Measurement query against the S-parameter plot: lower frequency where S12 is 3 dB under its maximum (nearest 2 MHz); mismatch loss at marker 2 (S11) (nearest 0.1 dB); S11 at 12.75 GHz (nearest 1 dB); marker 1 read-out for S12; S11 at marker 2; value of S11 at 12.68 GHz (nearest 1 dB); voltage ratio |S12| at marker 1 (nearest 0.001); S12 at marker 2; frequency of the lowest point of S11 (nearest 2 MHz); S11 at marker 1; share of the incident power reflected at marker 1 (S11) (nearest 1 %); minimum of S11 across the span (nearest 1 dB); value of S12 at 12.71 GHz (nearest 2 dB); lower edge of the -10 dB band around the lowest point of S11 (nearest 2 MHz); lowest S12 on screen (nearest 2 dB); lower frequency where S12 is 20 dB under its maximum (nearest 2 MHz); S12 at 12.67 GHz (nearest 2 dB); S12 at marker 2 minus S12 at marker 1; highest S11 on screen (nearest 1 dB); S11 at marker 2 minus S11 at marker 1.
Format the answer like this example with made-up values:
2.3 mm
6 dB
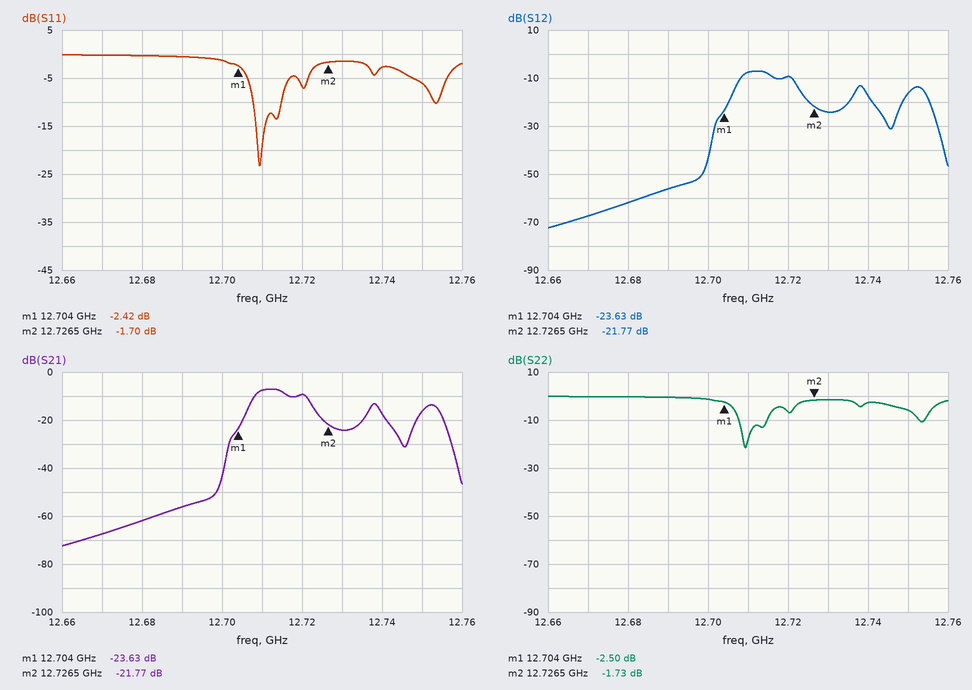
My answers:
12.708 GHz
4.9 dB
-6 dB
-23.63 dB
-1.70 dB
0 dB
0.066
-21.77 dB
12.710 GHz
-2.42 dB
57 %
-23 dB
-8 dB
12.708 GHz
-72 dB
12.702 GHz
-68 dB
1.86 dB
0 dB
0.72 dB
